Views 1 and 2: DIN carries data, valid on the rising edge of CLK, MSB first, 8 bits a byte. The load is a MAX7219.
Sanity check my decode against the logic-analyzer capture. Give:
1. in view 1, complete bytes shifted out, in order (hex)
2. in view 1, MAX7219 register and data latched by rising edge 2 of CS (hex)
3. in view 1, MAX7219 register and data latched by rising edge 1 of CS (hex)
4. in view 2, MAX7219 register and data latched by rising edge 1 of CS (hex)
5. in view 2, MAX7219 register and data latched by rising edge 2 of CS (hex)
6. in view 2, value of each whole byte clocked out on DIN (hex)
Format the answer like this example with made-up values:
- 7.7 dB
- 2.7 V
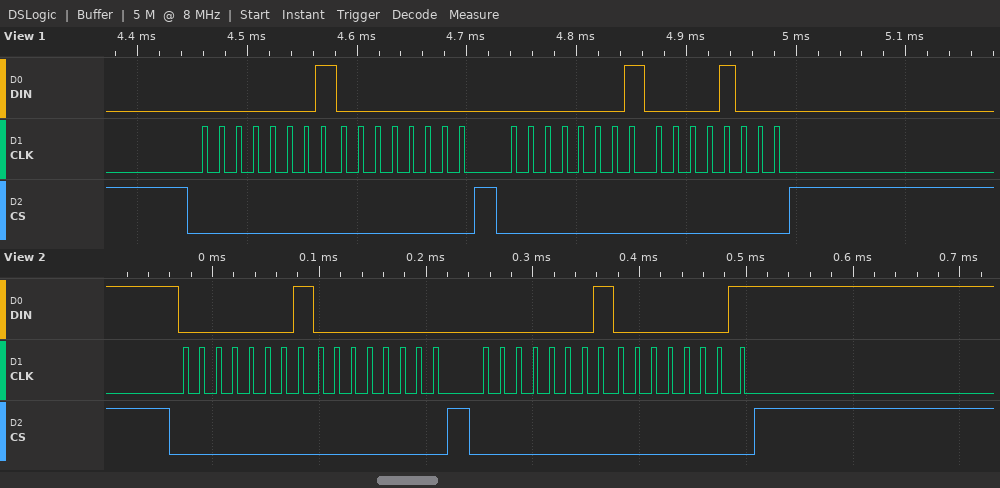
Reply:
- 01 00 01 08
- register 0x1, data 0x08
- register 0x1, data 0x00
- register 0x1, data 0x00
- register 0x1, data 0x01
- 01 00 01 01
